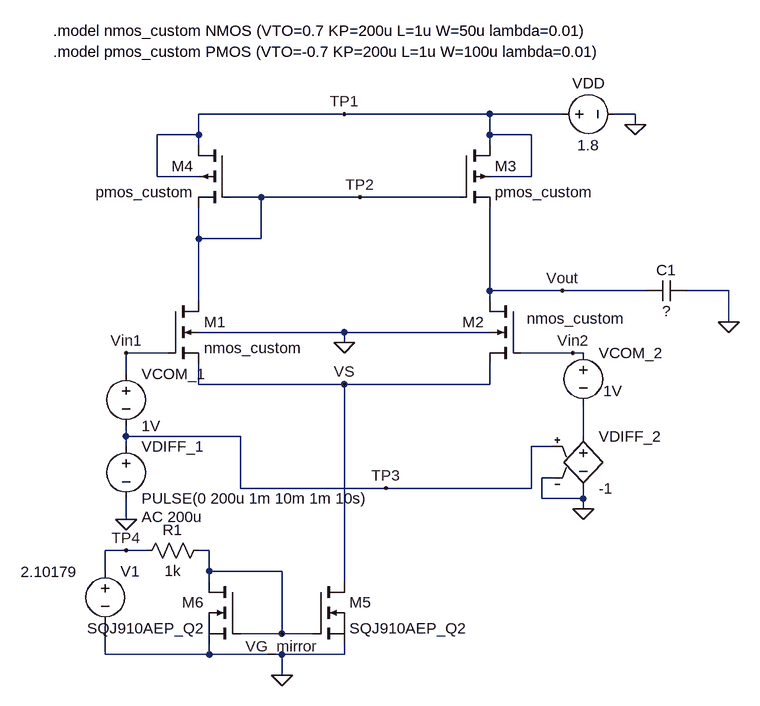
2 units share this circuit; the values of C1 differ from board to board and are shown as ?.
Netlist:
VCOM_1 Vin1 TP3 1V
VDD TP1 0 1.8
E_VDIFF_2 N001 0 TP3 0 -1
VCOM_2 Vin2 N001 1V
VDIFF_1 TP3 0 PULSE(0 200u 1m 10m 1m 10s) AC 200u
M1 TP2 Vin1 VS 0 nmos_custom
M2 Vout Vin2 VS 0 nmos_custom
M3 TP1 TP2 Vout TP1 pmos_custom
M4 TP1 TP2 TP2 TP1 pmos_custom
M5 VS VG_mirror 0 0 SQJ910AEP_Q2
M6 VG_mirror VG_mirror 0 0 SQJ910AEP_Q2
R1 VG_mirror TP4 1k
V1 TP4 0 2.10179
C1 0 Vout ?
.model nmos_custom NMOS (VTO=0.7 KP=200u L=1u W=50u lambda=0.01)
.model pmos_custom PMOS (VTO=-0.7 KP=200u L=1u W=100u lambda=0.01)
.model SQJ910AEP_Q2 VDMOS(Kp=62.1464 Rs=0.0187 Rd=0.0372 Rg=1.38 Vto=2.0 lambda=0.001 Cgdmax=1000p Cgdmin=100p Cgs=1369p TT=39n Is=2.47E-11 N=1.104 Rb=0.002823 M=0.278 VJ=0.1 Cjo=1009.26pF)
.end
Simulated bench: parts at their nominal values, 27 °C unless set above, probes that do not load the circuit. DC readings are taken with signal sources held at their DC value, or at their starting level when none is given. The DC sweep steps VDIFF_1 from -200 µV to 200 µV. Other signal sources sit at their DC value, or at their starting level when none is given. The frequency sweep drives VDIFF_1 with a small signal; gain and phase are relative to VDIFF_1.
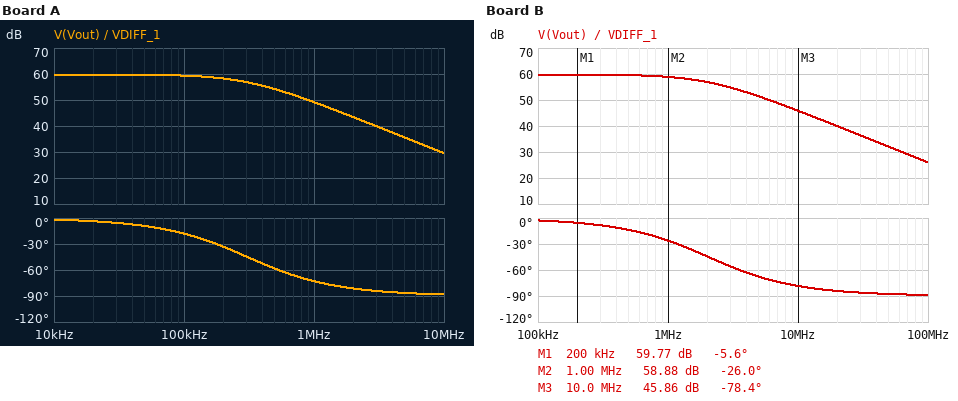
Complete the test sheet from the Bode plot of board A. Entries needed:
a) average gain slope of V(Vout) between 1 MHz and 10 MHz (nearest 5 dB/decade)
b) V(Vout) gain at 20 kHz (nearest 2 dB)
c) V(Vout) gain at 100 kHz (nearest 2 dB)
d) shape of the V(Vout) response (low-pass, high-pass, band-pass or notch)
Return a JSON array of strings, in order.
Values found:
["-20 dB/decade", "60 dB", "60 dB", "low-pass"]
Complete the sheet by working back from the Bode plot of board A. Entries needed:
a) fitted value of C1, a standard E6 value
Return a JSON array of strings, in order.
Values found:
["2.2 pF"]
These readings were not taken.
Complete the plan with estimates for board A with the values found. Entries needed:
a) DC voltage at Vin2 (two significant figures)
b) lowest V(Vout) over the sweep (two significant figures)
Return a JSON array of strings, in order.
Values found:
["1.0 V", "760 mV"]
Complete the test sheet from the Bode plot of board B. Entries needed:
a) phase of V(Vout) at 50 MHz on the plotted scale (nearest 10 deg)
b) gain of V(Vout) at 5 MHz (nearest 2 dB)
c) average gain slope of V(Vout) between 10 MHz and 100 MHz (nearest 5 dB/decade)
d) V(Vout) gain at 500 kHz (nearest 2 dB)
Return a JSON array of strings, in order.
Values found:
["-90 deg", "52 dB", "-20 dB/decade", "60 dB"]
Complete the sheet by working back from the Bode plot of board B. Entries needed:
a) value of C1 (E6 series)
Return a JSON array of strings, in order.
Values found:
["330 fF"]
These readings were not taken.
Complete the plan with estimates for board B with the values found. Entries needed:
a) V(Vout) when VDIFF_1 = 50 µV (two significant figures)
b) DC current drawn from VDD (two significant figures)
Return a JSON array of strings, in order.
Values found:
["1.0 V", "430 µA"]
